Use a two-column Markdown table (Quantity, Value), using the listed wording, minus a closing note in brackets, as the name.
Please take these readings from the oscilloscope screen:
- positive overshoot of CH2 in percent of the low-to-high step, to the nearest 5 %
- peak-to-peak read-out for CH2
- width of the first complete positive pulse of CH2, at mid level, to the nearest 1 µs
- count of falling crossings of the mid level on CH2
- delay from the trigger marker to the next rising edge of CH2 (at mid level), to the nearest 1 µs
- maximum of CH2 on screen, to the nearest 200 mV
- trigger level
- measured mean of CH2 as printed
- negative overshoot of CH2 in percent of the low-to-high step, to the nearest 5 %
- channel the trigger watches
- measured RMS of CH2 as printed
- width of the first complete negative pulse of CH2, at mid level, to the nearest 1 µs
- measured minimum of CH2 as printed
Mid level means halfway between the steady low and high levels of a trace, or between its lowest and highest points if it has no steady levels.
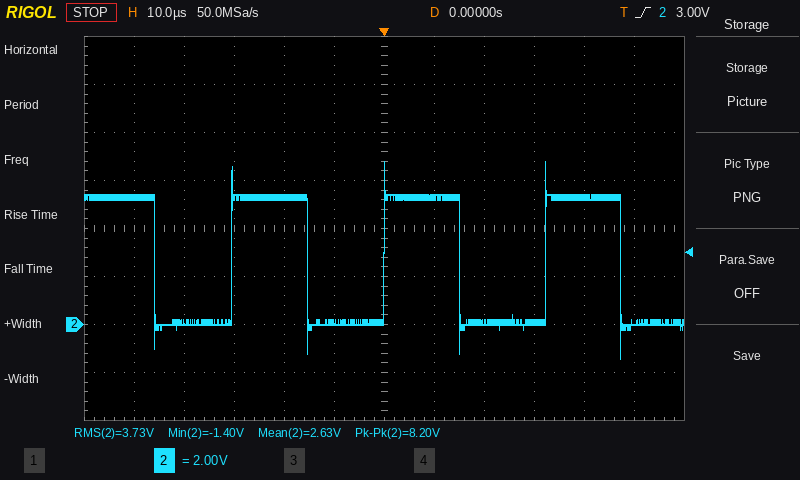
| Quantity | Value |
|---|---|
| positive overshoot of CH2 in percent of the low-to-high step, to the nearest 5 % | 30 % |
| peak-to-peak read-out for CH2 | 8.20 V |
| width of the first complete positive pulse of CH2, at mid level, to the nearest 1 µs | 15 µs |
| count of falling crossings of the mid level on CH2 | 4 |
| delay from the trigger marker to the next rising edge of CH2 (at mid level), to the nearest 1 µs | 32 µs |
| maximum of CH2 on screen, to the nearest 200 mV | 6.8 V |
| trigger level | 3.00 V |
| measured mean of CH2 as printed | 2.63 V |
| negative overshoot of CH2 in percent of the low-to-high step, to the nearest 5 % | 30 % |
| channel the trigger watches | CH2 |
| measured RMS of CH2 as printed | 3.73 V |
| width of the first complete negative pulse of CH2, at mid level, to the nearest 1 µs | 15 µs |
| measured minimum of CH2 as printed | -1.40 V |
